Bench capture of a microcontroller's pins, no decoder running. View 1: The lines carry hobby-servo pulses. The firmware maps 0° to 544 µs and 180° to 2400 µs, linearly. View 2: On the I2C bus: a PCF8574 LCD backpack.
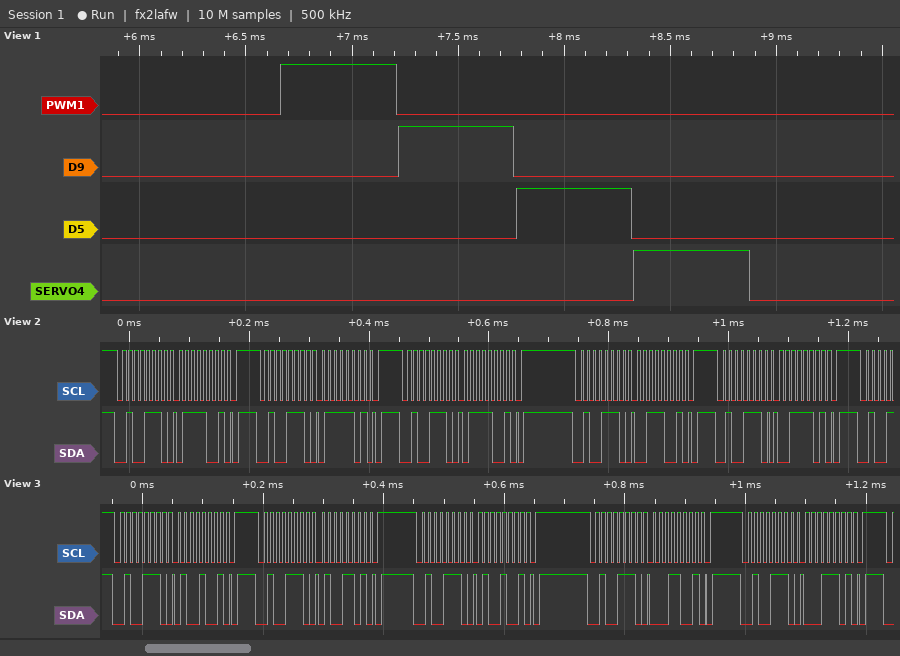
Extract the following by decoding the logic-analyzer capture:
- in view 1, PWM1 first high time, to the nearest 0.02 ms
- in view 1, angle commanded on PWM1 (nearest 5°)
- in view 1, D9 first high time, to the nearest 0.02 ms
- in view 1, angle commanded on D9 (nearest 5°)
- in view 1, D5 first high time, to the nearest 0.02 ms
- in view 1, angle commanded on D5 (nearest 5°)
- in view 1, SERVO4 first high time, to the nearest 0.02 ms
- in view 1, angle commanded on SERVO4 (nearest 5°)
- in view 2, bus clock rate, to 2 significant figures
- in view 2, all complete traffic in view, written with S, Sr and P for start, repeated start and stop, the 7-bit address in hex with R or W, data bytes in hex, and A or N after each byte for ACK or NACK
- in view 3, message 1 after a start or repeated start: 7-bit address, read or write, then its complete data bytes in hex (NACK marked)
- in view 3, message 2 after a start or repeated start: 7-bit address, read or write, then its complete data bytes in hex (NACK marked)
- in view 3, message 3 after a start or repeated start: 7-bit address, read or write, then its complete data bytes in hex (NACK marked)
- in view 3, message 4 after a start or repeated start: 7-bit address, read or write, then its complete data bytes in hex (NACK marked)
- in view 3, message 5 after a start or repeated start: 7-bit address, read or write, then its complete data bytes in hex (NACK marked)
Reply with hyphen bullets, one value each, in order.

- 0.54 ms
- 0°
- 0.54 ms
- 0°
- 0.54 ms
- 0°
- 0.54 ms
- 0°
- 100 kHz
- S 27W A 79 A P S 27W A 7D A P S 27W A 79 A P S 27W A 39 A P S 27W A 3D A P
- 0x27 write: 49
- 0x27 write: 4D
- 0x27 write: 49
- 0x27 write: 19
- 0x27 write: 1D
